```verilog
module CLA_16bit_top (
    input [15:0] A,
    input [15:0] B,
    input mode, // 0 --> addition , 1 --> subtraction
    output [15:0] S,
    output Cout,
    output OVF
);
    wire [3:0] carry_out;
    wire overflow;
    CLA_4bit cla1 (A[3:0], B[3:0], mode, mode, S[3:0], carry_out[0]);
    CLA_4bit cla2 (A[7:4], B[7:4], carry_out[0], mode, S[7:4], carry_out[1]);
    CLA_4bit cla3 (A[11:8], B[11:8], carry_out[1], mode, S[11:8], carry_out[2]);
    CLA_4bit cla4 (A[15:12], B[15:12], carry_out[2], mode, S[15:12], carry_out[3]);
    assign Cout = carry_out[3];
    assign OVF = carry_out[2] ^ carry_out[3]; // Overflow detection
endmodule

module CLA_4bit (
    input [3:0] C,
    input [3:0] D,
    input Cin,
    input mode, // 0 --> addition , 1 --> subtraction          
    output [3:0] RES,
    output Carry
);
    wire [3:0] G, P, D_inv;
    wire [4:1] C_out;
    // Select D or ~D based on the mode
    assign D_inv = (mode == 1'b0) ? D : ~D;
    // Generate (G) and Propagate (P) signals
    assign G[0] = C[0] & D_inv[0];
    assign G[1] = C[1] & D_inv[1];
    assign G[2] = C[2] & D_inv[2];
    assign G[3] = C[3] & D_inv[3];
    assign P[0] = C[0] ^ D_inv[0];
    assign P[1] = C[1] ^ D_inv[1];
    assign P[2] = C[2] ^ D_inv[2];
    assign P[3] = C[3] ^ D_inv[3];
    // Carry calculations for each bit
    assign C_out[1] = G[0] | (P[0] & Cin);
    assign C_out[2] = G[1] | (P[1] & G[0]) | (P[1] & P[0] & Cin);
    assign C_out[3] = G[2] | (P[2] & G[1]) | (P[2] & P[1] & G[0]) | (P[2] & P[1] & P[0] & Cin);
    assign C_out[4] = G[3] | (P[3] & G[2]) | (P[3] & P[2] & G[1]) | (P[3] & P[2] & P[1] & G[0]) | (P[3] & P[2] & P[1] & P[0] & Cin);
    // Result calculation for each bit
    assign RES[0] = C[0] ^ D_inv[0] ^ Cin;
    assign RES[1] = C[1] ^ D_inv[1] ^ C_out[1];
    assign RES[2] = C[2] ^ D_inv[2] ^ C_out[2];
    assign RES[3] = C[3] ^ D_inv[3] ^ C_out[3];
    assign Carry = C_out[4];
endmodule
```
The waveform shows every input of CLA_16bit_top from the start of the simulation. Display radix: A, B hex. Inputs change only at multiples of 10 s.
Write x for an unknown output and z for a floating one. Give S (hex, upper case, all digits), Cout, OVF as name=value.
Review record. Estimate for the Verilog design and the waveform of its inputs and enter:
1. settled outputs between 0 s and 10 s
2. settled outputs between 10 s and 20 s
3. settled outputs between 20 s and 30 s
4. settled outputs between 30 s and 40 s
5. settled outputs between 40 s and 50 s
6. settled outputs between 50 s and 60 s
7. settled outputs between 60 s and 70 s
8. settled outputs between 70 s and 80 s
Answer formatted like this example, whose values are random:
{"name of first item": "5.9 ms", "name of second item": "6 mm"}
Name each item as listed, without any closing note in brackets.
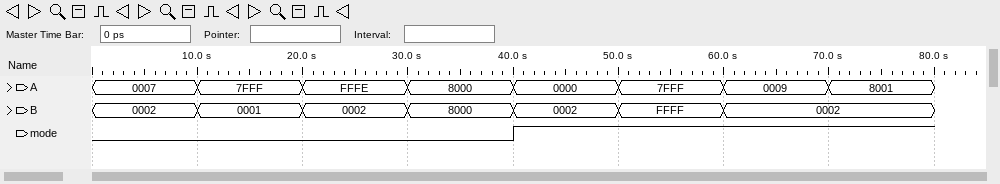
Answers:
{"settled outputs between 0 s and 10 s": "S=0009, Cout=0, OVF=0", "settled outputs between 10 s and 20 s": "S=8000, Cout=0, OVF=1", "settled outputs between 20 s and 30 s": "S=0000, Cout=1, OVF=0", "settled outputs between 30 s and 40 s": "S=0000, Cout=1, OVF=1", "settled outputs between 40 s and 50 s": "S=FFFE, Cout=0, OVF=0", "settled outputs between 50 s and 60 s": "S=8000, Cout=0, OVF=1", "settled outputs between 60 s and 70 s": "S=0007, Cout=1, OVF=0", "settled outputs between 70 s and 80 s": "S=7FFF, Cout=1, OVF=1"}
